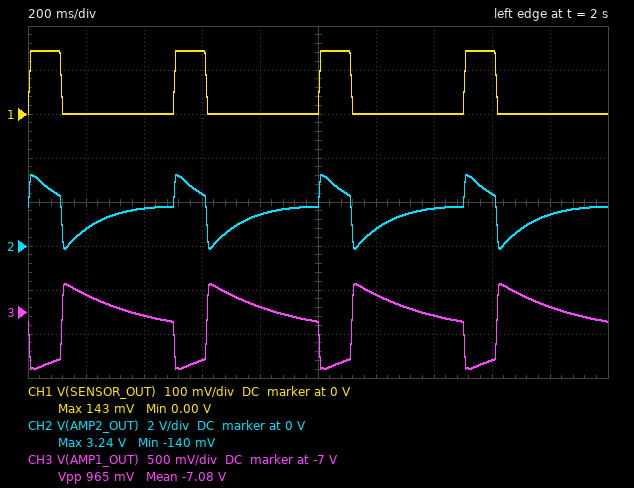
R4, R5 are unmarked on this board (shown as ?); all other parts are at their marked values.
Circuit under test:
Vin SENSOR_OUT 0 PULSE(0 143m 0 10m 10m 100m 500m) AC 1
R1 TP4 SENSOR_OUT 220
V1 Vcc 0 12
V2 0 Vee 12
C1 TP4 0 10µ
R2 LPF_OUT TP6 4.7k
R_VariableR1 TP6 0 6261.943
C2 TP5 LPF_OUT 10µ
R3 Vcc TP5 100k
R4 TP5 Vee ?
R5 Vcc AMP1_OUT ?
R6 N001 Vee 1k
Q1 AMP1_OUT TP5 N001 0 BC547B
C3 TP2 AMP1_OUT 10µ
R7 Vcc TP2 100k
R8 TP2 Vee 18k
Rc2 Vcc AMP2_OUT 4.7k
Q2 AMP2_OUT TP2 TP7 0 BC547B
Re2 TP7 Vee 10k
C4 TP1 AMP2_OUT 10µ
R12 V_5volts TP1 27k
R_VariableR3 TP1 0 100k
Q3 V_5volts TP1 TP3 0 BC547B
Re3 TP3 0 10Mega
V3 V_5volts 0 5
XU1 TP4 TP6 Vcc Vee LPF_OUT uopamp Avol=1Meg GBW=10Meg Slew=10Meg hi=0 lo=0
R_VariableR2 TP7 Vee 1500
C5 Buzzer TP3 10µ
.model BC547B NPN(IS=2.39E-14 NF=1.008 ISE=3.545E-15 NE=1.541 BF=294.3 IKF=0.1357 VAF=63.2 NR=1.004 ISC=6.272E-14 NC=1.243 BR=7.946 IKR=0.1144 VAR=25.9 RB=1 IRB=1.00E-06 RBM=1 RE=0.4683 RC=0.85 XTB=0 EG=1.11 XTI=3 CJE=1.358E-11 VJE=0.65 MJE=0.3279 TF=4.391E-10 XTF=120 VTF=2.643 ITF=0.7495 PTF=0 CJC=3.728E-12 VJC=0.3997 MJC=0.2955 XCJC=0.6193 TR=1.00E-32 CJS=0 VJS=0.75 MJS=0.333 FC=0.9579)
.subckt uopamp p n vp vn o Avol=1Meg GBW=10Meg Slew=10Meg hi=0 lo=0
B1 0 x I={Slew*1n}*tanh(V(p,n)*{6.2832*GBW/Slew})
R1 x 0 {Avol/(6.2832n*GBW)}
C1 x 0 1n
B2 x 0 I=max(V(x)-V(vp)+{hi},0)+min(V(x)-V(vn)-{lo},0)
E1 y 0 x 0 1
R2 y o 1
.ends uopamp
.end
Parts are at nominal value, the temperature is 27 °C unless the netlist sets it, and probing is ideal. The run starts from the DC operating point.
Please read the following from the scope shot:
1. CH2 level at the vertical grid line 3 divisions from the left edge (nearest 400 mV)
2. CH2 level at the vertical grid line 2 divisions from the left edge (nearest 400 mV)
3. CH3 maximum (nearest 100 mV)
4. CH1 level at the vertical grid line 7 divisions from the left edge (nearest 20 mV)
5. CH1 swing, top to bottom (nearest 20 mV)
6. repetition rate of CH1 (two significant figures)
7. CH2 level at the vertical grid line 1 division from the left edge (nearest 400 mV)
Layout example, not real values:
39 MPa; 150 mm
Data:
2.4 V; 1.6 V; -6.7 V; 0 V; 140 mV; 2.0 Hz; 800 mV
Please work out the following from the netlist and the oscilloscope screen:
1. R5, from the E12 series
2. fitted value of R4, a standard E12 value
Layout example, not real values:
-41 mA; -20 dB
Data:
4.7 kΩ; 27 kΩ
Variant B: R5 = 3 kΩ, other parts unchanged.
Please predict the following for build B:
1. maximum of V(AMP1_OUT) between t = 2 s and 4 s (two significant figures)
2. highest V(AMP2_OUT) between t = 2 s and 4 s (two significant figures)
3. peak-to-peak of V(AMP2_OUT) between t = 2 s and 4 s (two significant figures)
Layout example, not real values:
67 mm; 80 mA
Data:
-150 mV; 3.2 V; 2.8 V
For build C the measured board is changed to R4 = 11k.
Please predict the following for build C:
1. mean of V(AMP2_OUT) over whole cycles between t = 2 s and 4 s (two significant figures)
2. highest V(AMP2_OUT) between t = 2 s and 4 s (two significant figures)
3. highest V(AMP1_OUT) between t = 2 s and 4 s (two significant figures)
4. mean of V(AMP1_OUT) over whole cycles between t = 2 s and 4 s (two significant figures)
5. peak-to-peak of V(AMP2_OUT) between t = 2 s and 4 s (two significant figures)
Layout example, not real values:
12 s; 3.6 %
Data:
1.6 V; 3.5 V; 4.6 V; 4.1 V; 3.9 V
